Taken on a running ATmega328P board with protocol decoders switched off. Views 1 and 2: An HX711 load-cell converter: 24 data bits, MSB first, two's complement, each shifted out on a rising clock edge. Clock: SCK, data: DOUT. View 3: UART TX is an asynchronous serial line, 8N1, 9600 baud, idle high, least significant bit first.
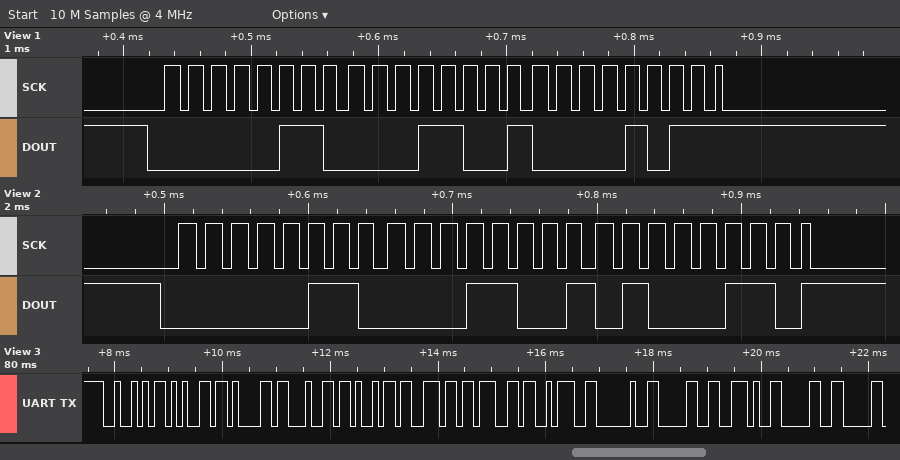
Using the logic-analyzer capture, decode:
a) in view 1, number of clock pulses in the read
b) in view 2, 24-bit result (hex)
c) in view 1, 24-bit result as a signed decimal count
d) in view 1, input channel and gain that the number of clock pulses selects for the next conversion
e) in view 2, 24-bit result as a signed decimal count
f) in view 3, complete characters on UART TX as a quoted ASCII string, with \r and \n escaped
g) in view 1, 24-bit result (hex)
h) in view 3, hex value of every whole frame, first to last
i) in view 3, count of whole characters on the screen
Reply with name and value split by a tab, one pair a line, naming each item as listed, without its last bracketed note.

in view 1, number of clock pulses in the read	25
in view 2, 24-bit result	0x061946
in view 1, 24-bit result as a signed decimal count	399627
in view 1, input channel and gain that the number of clock pulses selects for the next conversion	channel A, gain 128
in view 2, 24-bit result as a signed decimal count	399686
in view 3, complete characters on UART TX as a quoted ASCII string, with \r and \n escaped	"Reading: 0.0"
in view 1, 24-bit result	0x06190B
in view 3, hex value of every whole frame, first to last	52 65 61 64 69 6E 67 3A 20 30 2E 30
in view 3, count of whole characters on the screen	12
